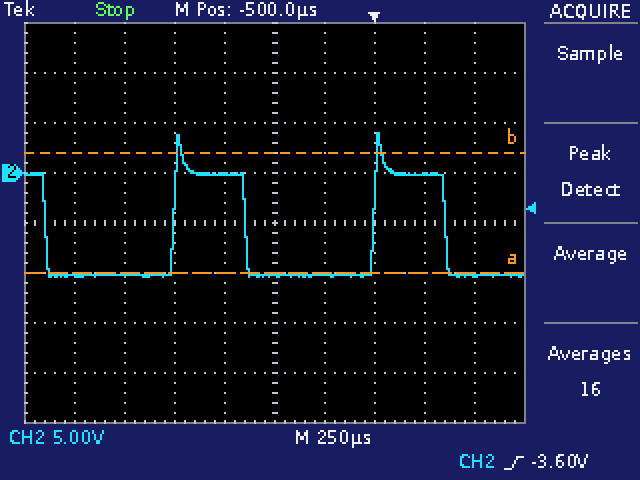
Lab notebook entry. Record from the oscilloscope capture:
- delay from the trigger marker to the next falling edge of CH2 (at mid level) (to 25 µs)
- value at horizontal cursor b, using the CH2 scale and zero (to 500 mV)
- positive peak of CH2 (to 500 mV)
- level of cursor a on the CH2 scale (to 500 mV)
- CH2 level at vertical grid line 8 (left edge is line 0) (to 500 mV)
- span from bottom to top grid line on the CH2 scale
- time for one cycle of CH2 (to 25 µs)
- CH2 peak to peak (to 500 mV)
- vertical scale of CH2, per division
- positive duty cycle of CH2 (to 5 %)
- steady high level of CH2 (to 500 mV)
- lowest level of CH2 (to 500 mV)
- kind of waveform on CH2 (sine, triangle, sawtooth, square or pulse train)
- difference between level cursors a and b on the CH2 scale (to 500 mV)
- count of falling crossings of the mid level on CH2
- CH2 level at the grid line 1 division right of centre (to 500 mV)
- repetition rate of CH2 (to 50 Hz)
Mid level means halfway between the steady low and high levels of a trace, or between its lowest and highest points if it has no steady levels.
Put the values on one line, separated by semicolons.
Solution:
350 µs; 2.0 V; 4.0 V; -10.0 V; 0.0 V; 40 V; 1.000 ms; 14.5 V; 5 V; 35 %; 0.0 V; -10.5 V; pulse train; 12.0 V; 3; -10.0 V; 1.00 kHz
